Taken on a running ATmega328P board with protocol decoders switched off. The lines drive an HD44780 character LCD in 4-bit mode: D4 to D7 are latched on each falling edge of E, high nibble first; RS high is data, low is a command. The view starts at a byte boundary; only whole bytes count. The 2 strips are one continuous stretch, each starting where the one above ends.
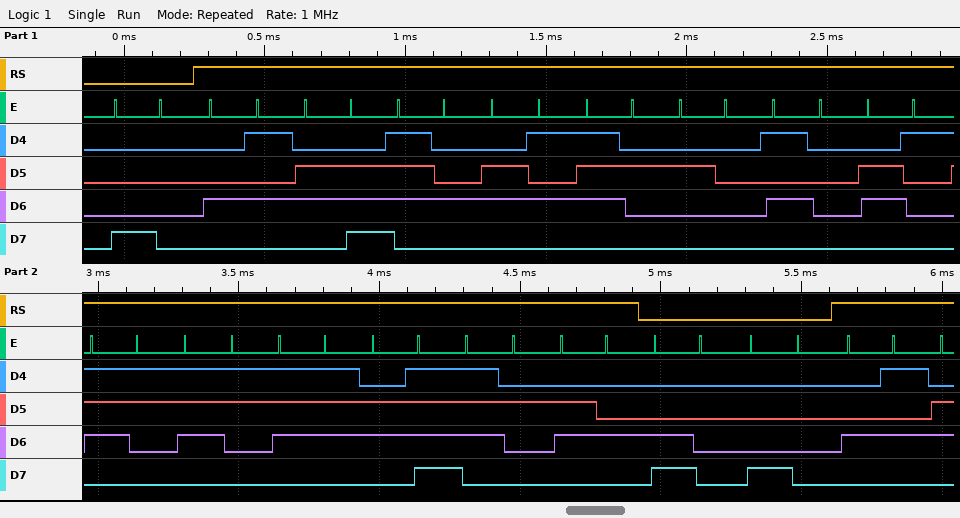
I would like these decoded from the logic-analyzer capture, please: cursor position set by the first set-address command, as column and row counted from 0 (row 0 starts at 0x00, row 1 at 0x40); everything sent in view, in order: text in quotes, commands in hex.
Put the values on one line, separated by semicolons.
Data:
column 0, row 0; 0x80 "Enter Password" 0xC0 0x80 "E"
